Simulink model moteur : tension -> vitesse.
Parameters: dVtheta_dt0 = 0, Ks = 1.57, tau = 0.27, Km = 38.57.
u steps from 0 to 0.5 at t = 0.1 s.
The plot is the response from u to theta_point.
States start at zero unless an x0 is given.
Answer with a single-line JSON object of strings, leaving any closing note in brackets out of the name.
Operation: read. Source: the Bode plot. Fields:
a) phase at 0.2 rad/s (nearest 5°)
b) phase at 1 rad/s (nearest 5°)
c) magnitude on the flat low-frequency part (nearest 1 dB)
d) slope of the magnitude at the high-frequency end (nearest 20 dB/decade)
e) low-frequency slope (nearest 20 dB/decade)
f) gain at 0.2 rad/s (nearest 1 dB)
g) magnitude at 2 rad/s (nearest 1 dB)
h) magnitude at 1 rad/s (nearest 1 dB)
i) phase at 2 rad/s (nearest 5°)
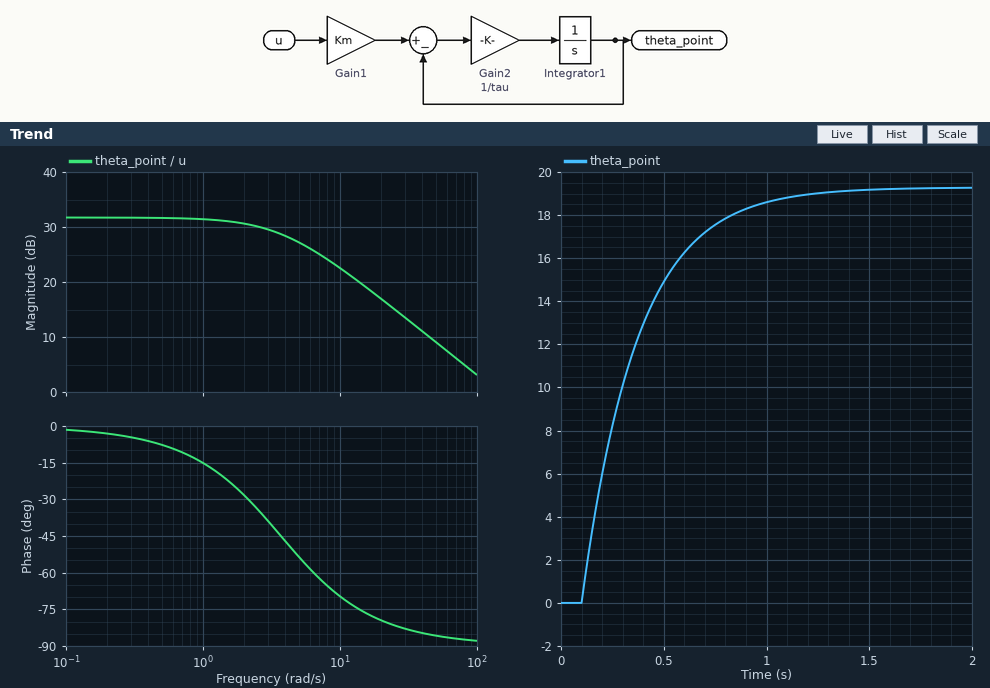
{"phase at 0.2 rad/s": "-5°", "phase at 1 rad/s": "-15°", "magnitude on the flat low-frequency part": "32 dB", "slope of the magnitude at the high-frequency end": "-20 dB/decade", "low-frequency slope": "0 dB/decade", "gain at 0.2 rad/s": "32 dB", "magnitude at 2 rad/s": "31 dB", "magnitude at 1 rad/s": "31 dB", "phase at 2 rad/s": "-30°"}
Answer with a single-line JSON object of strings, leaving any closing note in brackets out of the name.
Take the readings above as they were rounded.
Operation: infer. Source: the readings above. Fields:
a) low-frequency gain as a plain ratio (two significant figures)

{"low-frequency gain as a plain ratio": "40"}
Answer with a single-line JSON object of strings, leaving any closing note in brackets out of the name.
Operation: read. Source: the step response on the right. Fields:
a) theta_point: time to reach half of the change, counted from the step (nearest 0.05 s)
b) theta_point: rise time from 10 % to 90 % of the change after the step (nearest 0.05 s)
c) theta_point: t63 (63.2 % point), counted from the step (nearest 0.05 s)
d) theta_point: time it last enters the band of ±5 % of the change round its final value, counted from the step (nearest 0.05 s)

{"theta_point: time to reach half of the change, counted from the step": "0.20 s", "theta_point: rise time from 10 % to 90 % of the change after the step": "0.60 s", "theta_point: t63 (63.2 % point), counted from the step": "0.25 s", "theta_point: time it last enters the band of ±5 % of the change round its final value, counted from the step": "0.80 s"}
